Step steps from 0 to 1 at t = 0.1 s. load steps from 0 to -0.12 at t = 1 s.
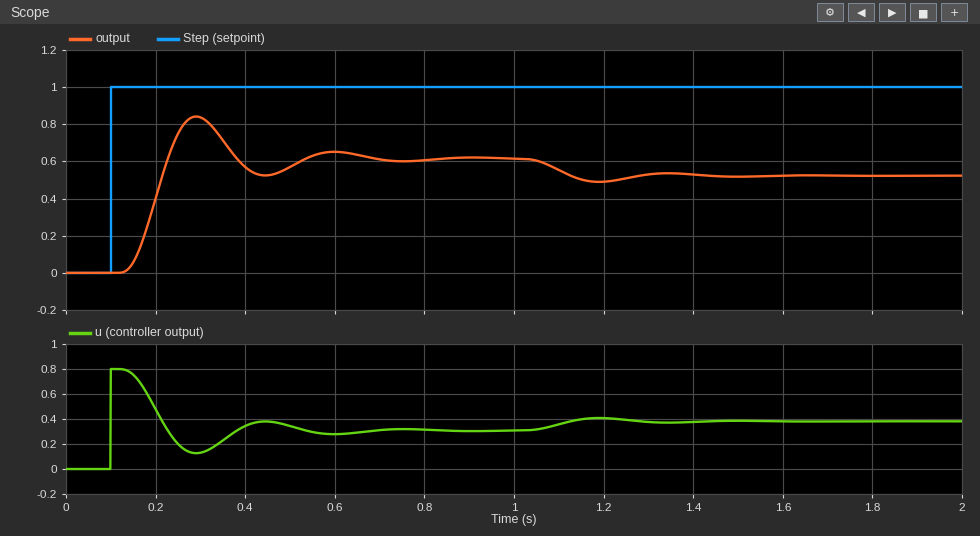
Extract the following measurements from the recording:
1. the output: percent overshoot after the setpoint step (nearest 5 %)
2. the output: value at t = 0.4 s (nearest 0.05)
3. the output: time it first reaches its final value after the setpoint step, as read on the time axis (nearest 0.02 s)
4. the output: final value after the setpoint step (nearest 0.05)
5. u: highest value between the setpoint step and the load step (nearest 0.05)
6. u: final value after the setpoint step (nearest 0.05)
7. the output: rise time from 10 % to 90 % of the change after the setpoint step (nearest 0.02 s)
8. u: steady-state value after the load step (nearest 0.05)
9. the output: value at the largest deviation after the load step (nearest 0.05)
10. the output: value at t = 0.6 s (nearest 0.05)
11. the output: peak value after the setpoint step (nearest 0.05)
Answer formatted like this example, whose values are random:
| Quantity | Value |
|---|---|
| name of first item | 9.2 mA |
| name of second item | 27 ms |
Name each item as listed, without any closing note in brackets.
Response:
| Quantity | Value |
|---|---|
| the output: percent overshoot after the setpoint step | 35 % |
| the output: value at t = 0.4 s | 0.55 |
| the output: time it first reaches its final value after the setpoint step, as read on the time axis | 0.22 s |
| the output: final value after the setpoint step | 0.60 |
| u: highest value between the setpoint step and the load step | 0.80 |
| u: final value after the setpoint step | 0.30 |
| the output: rise time from 10 % to 90 % of the change after the setpoint step | 0.06 s |
| u: steady-state value after the load step | 0.40 |
| the output: value at the largest deviation after the load step | 0.50 |
| the output: value at t = 0.6 s | 0.65 |
| the output: peak value after the setpoint step | 0.85 |
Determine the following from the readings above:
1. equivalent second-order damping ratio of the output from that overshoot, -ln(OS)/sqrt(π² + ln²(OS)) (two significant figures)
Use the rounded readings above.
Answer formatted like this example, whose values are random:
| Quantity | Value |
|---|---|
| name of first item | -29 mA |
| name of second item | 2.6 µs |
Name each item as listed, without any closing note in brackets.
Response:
| Quantity | Value |
|---|---|
| equivalent second-order damping ratio of the output from that overshoot, -ln(OS)/sqrt(π² + ln²(OS)) | 0.32 |
